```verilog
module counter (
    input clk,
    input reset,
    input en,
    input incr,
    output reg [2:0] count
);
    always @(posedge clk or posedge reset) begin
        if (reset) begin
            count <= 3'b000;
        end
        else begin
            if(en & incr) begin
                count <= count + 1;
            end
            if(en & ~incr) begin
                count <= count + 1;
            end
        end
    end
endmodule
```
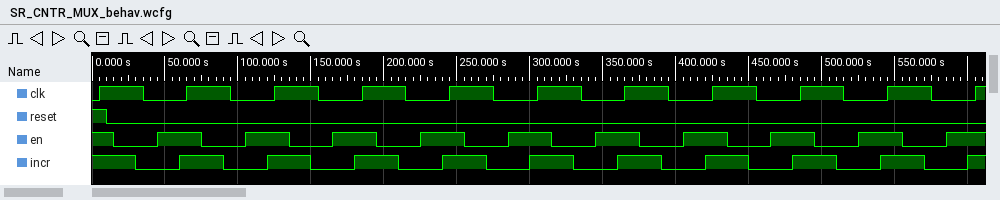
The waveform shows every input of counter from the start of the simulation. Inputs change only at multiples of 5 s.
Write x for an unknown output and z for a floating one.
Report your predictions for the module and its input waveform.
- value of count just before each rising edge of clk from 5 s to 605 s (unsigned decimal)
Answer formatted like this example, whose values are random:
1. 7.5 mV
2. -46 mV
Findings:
1. 0, 0, 1, 2, 3, 4, 5, 6, 7, 0, 1
